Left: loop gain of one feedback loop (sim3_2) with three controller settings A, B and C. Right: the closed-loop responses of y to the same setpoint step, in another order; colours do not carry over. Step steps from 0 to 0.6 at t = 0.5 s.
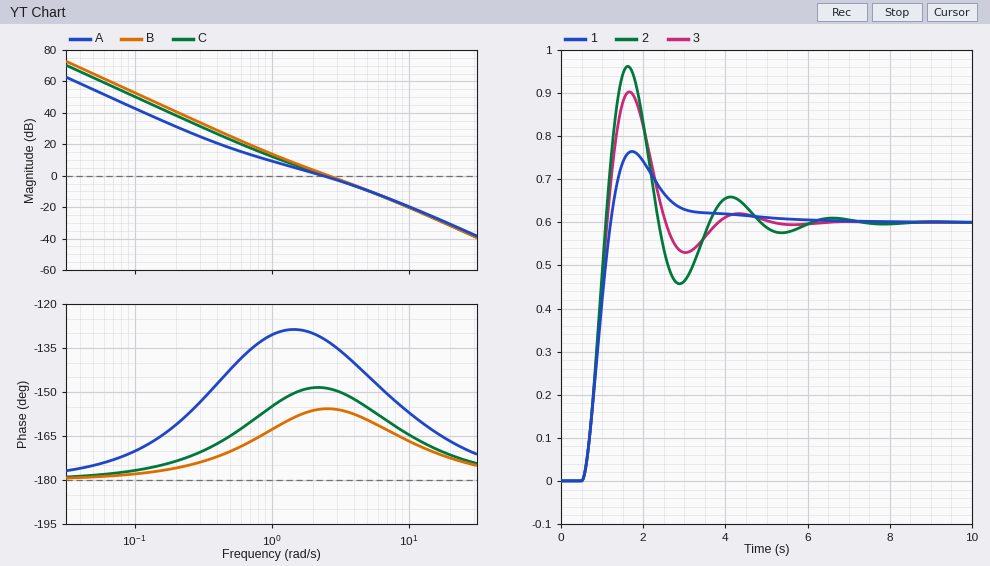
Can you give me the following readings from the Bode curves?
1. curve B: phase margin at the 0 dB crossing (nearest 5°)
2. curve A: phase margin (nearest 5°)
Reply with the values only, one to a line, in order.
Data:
25°
50°
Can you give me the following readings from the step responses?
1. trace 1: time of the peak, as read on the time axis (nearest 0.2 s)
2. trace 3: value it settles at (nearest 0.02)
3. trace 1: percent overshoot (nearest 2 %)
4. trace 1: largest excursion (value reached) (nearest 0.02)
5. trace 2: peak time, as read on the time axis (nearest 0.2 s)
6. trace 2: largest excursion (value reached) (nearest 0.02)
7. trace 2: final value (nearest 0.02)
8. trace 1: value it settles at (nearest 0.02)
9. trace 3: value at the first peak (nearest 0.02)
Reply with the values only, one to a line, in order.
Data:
1.8 s
0.60
28 %
0.76
1.6 s
0.96
0.60
0.60
0.90
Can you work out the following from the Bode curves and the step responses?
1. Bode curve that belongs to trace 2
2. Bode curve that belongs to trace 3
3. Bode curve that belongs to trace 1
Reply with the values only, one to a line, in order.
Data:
B
C
A
